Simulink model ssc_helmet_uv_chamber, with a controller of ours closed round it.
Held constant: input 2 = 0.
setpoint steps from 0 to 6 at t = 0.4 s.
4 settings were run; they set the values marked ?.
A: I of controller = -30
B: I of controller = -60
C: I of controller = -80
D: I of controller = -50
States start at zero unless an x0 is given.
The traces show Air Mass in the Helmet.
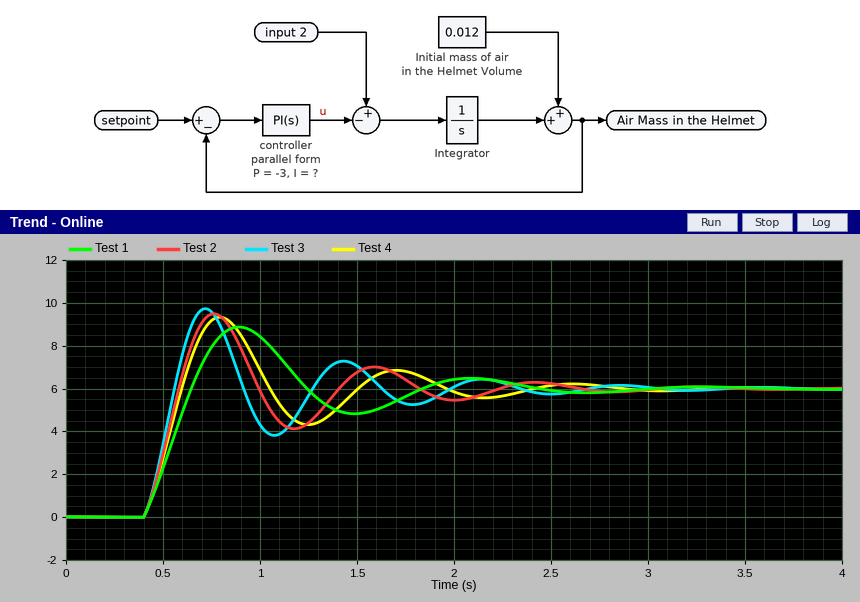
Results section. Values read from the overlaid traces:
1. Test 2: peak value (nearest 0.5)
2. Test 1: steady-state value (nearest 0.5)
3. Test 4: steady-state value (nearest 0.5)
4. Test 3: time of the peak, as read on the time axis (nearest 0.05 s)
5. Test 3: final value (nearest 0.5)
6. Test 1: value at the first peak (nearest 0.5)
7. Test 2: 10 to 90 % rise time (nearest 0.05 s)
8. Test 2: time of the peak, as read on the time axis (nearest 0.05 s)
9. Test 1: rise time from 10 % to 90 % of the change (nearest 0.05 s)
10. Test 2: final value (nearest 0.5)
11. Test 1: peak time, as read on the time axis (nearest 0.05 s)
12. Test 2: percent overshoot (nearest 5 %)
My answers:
9.5
6.0
6.0
0.70 s
6.0
9.0
0.15 s
0.75 s
0.20 s
6.0
0.90 s
60 %
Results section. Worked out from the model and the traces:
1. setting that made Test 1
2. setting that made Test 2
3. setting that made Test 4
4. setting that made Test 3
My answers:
A
B
D
C
